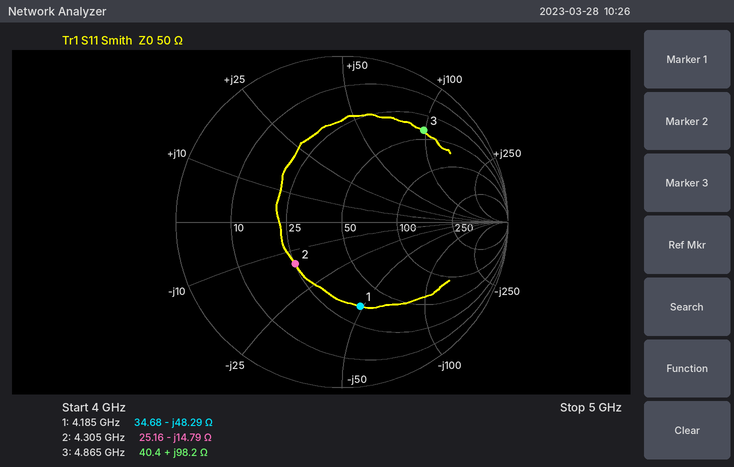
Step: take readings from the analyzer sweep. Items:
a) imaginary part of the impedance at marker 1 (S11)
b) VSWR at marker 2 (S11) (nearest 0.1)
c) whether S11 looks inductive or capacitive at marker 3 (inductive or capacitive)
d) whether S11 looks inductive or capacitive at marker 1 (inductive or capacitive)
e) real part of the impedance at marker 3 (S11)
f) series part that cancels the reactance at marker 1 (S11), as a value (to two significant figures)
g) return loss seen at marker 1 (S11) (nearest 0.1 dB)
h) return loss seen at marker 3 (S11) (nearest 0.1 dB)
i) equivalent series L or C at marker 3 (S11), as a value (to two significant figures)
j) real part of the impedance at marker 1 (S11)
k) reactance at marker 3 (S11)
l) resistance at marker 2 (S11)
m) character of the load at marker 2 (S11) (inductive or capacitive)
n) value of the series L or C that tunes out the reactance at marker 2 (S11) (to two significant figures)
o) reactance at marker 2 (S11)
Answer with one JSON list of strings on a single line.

["-48.29 Ω", "2.2", "inductive", "capacitive", "40.4 Ω", "1.8 nH", "5.7 dB", "2.6 dB", "3.2 nH", "34.68 Ω", "+98.2 Ω", "25.16 Ω", "capacitive", "550 pH", "-14.79 Ω"]
